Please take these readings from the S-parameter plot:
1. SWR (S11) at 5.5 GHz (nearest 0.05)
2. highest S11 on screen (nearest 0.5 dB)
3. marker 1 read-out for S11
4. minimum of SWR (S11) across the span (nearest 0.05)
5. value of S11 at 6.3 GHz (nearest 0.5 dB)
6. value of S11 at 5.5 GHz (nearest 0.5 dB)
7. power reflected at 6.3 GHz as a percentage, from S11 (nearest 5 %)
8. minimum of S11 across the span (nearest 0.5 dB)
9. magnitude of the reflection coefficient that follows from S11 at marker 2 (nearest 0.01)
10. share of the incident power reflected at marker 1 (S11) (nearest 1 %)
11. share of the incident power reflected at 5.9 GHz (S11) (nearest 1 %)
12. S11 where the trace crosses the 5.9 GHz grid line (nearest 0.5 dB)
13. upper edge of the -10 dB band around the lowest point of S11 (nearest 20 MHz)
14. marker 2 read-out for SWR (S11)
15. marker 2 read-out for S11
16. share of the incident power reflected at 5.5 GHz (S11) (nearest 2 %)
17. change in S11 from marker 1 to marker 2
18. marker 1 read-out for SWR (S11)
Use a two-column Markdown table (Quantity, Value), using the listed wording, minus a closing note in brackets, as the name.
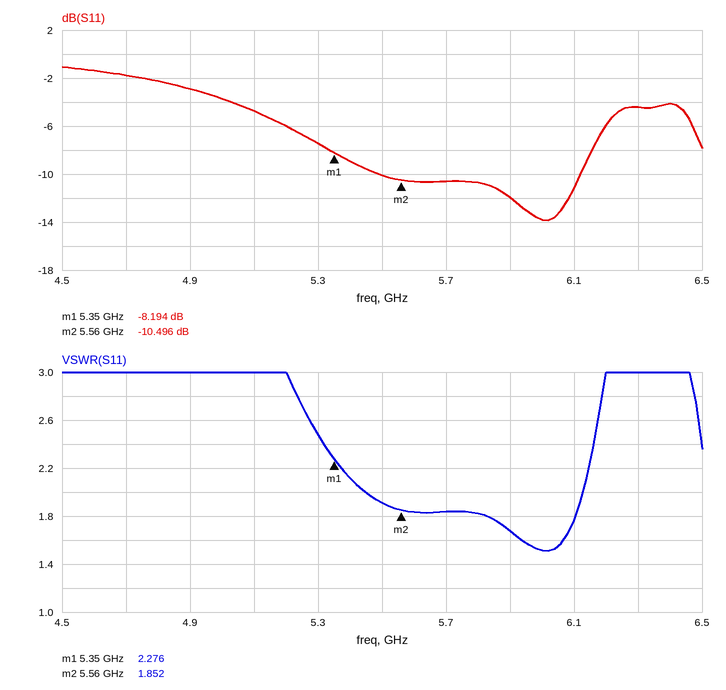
| Quantity | Value |
|---|---|
| SWR (S11) at 5.5 GHz | 1.90 |
| highest S11 on screen | -1.0 dB |
| marker 1 read-out for S11 | -8.194 dB |
| minimum of SWR (S11) across the span | 1.50 |
| value of S11 at 6.3 GHz | -4.5 dB |
| value of S11 at 5.5 GHz | -10.0 dB |
| power reflected at 6.3 GHz as a percentage, from S11 | 35 % |
| minimum of S11 across the span | -14.0 dB |
| magnitude of the reflection coefficient that follows from S11 at marker 2 | 0.30 |
| share of the incident power reflected at marker 1 (S11) | 15 % |
| share of the incident power reflected at 5.9 GHz (S11) | 6 % |
| S11 where the trace crosses the 5.9 GHz grid line | -12.0 dB |
| upper edge of the -10 dB band around the lowest point of S11 | 6.12 GHz |
| marker 2 read-out for SWR | 1.852 |
| marker 2 read-out for S11 | -10.496 dB |
| share of the incident power reflected at 5.5 GHz (S11) | 10 % |
| change in S11 from marker 1 to marker 2 | -2.302 dB |
| marker 1 read-out for SWR | 2.276 |
